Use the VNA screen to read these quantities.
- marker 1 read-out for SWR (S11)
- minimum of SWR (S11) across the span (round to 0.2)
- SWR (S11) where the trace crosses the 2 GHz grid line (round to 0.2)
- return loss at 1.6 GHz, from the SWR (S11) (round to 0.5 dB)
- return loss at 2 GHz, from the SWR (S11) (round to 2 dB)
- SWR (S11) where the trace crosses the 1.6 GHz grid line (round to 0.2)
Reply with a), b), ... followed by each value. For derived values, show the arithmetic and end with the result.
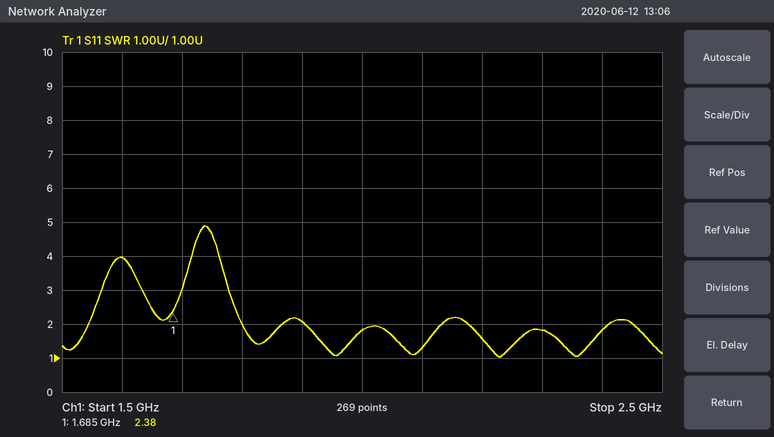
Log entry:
a) 2.38
b) 1.0
c) 1.8
d) −20 log10((4 − 1)/(4 + 1)) ≈ 4.44 dB, so 4.5 dB to the nearest 0.5 dB
e) −20 log10((1.8 − 1)/(1.8 + 1)) ≈ 10.9 dB, so 10 dB to the nearest 2 dB
f) 4.0
